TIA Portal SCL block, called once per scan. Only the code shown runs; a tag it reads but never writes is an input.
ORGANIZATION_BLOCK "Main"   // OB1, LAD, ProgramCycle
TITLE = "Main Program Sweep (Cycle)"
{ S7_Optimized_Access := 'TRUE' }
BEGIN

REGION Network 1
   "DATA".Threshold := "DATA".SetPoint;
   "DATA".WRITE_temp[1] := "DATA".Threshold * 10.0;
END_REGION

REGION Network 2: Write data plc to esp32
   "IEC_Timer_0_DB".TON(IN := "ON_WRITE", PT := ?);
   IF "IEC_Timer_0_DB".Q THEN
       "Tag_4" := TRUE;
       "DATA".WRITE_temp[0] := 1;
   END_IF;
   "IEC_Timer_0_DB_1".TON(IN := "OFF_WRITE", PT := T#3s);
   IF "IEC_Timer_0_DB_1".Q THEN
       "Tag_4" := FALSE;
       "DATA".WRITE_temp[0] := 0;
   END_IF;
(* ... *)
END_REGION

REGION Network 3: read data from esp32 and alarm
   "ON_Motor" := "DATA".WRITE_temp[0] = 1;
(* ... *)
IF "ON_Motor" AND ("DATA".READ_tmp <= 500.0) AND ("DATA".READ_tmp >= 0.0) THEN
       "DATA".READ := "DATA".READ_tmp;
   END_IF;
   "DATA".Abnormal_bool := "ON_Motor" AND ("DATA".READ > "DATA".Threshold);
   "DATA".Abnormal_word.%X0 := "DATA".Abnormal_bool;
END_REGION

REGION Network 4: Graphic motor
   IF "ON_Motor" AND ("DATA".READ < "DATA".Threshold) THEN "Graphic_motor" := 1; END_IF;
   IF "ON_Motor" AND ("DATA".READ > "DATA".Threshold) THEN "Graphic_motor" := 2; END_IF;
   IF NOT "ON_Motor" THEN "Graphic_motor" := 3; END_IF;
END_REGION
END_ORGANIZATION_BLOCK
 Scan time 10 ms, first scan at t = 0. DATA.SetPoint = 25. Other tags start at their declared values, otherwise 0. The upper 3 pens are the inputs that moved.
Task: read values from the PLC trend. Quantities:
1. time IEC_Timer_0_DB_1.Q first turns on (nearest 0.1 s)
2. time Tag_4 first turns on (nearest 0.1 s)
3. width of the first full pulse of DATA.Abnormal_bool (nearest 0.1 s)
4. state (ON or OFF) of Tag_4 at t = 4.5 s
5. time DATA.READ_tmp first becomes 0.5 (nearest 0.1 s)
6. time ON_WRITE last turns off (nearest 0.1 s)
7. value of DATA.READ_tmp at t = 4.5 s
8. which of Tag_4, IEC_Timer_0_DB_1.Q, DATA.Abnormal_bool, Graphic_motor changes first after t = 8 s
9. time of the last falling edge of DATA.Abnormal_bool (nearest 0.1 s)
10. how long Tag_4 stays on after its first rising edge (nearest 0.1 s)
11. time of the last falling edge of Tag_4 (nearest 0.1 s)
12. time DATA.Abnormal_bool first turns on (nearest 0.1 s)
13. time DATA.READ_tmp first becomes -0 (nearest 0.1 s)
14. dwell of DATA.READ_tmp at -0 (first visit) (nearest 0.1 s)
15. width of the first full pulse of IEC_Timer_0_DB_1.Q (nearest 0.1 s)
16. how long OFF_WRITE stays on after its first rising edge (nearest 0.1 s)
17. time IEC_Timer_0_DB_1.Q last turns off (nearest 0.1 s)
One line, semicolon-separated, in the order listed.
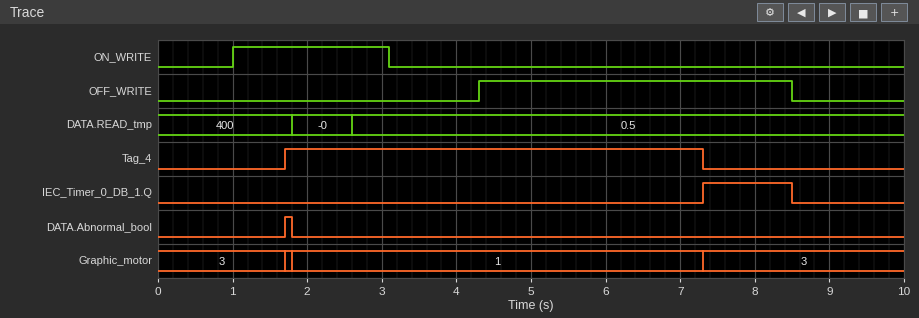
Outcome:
7.3 s; 1.7 s; 0.1 s; ON; 2.6 s; 3.1 s; 0.5; IEC_Timer_0_DB_1.Q; 1.8 s; 5.6 s; 7.3 s; 1.7 s; 1.8 s; 0.8 s; 1.2 s; 4.2 s; 8.5 s
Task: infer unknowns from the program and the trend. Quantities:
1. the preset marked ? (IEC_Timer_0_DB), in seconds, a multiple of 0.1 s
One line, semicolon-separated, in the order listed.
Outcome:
0.7 s
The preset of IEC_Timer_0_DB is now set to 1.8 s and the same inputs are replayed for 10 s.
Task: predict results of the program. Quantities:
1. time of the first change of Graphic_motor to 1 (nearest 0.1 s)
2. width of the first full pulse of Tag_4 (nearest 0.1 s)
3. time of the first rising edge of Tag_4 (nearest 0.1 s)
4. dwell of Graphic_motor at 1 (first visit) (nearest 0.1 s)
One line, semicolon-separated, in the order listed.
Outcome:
2.8 s; 4.5 s; 2.8 s; 4.5 s
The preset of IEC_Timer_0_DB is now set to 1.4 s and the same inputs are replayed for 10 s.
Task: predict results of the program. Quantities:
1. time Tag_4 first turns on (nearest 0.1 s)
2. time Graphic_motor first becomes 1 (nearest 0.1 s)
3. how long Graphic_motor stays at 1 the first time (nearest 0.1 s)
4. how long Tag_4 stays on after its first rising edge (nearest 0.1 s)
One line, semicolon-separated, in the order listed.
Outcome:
2.4 s; 2.4 s; 4.9 s; 4.9 s
